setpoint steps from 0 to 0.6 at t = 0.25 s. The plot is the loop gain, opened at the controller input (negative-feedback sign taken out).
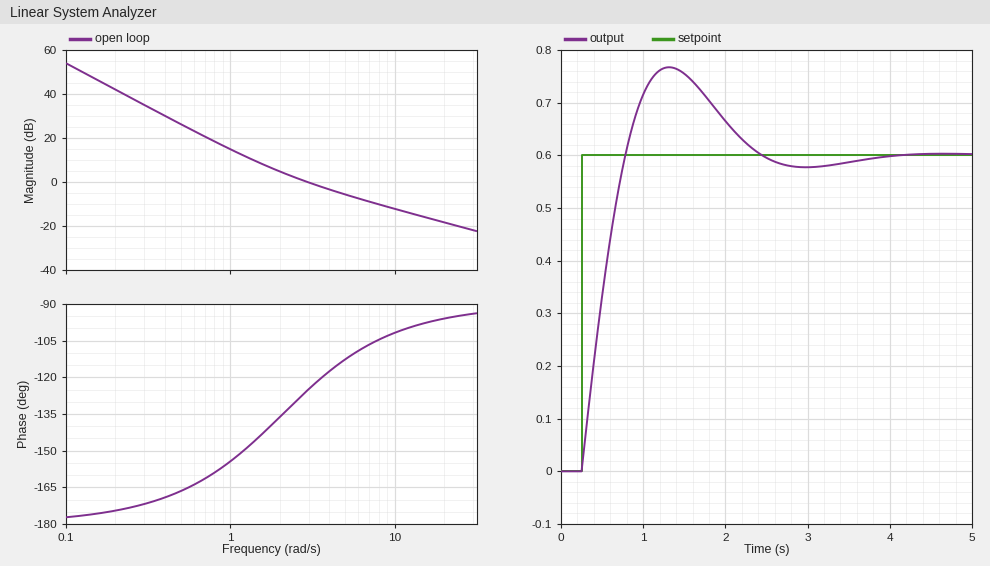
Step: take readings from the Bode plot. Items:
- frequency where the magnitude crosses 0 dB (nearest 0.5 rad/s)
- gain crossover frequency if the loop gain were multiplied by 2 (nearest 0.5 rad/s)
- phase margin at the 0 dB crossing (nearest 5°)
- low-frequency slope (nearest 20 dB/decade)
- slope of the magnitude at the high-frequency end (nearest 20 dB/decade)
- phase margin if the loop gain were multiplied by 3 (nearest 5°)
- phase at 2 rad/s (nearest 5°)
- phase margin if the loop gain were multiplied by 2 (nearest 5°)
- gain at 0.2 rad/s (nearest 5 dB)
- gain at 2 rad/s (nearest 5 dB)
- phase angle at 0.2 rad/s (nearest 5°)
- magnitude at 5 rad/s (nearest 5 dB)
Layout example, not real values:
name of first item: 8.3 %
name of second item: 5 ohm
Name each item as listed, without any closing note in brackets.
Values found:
frequency where the magnitude crosses 0 dB: 3.0 rad/s
gain crossover frequency if the loop gain were multiplied by 2: 5.0 rad/s
phase margin at the 0 dB crossing: 55°
low-frequency slope: -40 dB/decade
slope of the magnitude at the high-frequency end: -20 dB/decade
phase margin if the loop gain were multiplied by 3: 75°
phase at 2 rad/s: -135°
phase margin if the loop gain were multiplied by 2: 70°
gain at 0.2 rad/s: 40 dB
gain at 2 rad/s: 5 dB
phase angle at 0.2 rad/s: -175°
magnitude at 5 rad/s: -5 dB
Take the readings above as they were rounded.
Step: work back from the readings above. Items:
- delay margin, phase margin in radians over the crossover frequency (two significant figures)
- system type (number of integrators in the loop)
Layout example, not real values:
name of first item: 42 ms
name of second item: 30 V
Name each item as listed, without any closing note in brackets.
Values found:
delay margin, phase margin in radians over the crossover frequency: 0.32 s
system type: 2
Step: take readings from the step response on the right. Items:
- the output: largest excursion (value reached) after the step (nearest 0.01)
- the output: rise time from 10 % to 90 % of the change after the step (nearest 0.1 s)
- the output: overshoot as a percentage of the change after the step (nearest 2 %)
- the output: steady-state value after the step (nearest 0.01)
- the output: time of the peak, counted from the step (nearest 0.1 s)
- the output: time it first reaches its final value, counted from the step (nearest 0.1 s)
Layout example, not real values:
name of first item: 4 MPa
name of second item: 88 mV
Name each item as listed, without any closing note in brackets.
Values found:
the output: largest excursion (value reached) after the step: 0.77
the output: rise time from 10 % to 90 % of the change after the step: 0.4 s
the output: overshoot as a percentage of the change after the step: 28 %
the output: steady-state value after the step: 0.60
the output: time of the peak, counted from the step: 1.1 s
the output: time it first reaches its final value, counted from the step: 0.5 s
